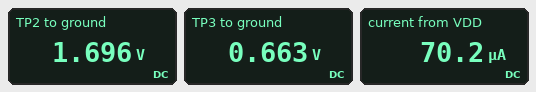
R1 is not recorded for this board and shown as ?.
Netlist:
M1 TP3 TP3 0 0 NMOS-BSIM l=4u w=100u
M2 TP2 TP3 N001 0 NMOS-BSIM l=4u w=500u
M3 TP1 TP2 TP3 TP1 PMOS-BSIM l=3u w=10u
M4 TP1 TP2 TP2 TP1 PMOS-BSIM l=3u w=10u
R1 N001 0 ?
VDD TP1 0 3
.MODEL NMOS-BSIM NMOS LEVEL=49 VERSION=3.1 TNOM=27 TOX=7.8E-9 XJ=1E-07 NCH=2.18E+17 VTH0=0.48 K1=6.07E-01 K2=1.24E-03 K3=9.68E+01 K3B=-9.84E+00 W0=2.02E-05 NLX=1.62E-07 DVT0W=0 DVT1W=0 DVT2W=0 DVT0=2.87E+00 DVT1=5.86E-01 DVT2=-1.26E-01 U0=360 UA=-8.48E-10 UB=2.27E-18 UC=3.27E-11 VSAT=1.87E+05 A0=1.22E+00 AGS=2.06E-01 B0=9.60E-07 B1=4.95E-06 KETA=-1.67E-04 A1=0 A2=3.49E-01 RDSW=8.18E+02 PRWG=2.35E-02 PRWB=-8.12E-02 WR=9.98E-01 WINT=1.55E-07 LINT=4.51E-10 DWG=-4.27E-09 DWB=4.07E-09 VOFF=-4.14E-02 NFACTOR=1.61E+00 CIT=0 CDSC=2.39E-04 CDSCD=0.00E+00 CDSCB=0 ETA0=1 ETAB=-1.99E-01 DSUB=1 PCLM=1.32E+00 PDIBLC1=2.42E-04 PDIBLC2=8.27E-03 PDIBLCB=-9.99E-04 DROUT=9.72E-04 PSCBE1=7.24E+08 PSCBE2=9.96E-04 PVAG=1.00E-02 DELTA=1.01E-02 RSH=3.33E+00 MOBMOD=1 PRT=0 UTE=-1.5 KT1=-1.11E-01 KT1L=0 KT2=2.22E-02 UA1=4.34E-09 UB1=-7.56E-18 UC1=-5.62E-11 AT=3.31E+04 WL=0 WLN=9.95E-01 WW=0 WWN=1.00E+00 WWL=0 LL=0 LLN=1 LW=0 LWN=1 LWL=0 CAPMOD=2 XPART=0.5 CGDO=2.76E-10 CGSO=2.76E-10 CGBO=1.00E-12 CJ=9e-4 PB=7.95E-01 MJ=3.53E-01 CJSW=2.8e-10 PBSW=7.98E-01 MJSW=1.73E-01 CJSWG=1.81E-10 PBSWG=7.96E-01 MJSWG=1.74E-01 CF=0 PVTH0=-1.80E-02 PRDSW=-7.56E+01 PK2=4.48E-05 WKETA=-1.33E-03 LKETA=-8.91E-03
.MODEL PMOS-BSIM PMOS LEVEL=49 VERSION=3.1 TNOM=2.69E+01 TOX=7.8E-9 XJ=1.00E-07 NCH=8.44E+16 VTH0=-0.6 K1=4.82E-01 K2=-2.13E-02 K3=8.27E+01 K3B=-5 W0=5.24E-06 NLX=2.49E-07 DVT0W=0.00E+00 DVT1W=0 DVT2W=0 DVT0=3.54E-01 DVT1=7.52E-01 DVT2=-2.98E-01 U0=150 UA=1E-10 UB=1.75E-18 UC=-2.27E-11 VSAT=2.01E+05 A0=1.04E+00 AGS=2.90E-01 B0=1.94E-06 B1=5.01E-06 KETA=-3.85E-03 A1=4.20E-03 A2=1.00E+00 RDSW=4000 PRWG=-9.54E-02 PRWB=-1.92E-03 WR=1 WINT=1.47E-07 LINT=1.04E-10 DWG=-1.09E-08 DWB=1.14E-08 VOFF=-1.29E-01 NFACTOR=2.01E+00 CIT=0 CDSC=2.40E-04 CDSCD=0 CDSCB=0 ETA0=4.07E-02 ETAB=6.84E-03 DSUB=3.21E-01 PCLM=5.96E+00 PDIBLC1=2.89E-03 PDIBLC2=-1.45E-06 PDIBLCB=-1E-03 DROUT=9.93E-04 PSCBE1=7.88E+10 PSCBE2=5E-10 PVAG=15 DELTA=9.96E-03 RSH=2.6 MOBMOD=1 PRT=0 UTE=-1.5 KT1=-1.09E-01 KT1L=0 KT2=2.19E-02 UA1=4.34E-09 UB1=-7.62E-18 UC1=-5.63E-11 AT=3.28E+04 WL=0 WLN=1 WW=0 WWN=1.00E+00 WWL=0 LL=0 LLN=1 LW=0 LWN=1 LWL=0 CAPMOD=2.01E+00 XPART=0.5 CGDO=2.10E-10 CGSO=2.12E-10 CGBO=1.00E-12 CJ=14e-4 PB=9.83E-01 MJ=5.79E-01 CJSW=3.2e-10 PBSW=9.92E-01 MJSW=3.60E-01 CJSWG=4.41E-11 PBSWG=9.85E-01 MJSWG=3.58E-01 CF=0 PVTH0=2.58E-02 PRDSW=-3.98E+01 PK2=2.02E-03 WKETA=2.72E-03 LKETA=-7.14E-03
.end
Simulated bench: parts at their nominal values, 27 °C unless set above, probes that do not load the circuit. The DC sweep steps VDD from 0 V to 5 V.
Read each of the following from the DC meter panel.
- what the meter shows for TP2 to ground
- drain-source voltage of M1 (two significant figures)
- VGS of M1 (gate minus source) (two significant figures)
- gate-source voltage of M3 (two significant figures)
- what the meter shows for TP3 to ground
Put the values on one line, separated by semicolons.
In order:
1.696 V; 660 mV; 660 mV; 1.0 V; 0.663 V
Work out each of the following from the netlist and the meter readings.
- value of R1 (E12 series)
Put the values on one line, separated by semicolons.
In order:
2.2 kΩ
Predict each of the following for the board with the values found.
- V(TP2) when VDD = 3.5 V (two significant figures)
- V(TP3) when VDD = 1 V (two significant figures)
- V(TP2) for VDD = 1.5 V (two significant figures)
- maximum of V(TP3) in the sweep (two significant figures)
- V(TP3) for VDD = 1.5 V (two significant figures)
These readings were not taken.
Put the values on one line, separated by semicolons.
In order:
2.2 V; 580 mV; 230 mV; 670 mV; 650 mV
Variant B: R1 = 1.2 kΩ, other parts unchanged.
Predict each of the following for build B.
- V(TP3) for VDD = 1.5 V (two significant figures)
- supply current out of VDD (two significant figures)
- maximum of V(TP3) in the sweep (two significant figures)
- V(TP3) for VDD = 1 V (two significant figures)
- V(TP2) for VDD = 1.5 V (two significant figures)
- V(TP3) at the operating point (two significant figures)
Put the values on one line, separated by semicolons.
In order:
680 mV; 150 µA; 740 mV; 590 mV; 96 mV; 720 mV
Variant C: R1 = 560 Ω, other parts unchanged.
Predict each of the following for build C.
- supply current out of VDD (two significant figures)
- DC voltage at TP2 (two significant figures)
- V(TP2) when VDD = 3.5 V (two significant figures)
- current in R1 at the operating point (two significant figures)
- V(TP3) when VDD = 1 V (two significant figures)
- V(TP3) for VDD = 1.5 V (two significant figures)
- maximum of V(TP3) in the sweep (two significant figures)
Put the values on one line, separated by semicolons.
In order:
540 µA; 330 mV; 750 mV; 270 µA; 590 mV; 690 mV; 930 mV
